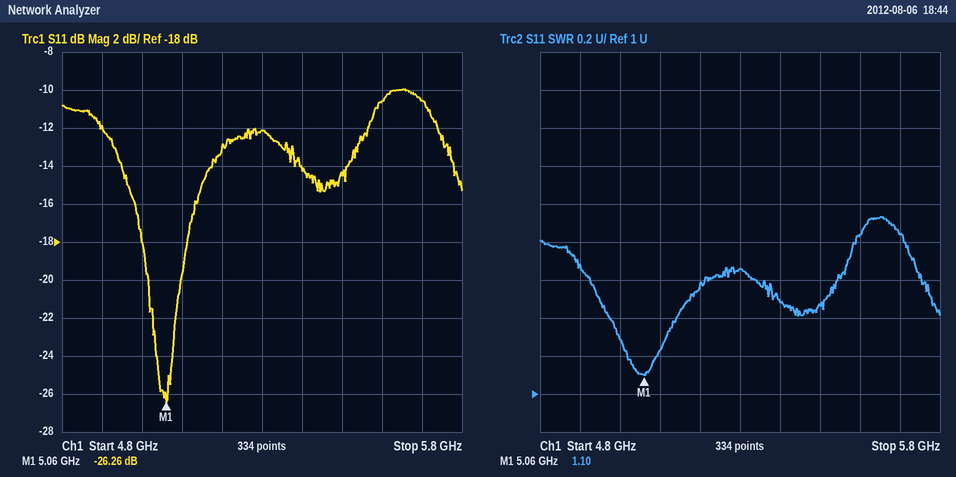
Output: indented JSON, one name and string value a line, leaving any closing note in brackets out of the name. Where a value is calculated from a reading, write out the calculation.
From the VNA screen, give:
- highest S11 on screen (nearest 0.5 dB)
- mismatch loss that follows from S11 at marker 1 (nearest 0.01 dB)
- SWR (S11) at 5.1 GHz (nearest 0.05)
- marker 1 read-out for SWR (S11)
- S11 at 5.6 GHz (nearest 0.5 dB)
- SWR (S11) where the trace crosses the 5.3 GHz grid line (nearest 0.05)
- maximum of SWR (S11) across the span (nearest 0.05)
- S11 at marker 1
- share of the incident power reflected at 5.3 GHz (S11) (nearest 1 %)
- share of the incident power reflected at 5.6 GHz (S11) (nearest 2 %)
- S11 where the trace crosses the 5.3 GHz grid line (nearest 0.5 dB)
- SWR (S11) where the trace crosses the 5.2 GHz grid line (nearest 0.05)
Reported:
{
  "highest S11 on screen": "-10.0 dB",
  "mismatch loss that follows from S11 at marker 1": "−10 log10(1 − 10^(-26.26/10)) ≈ 0.01 dB",
  "SWR (S11) at 5.1 GHz": "1.25",
  "marker 1 read-out for SWR": "1.10",
  "S11 at 5.6 GHz": "-10.5 dB",
  "SWR (S11) where the trace crosses the 5.3 GHz grid line": "1.65",
  "maximum of SWR (S11) across the span": "1.95",
  "S11 at marker 1": "-26.26 dB",
  "share of the incident power reflected at 5.3 GHz (S11)": "10^(-12/10) ≈ 6 %",
  "share of the incident power reflected at 5.6 GHz (S11)": "10^(-10.5/10) ≈ 8.91 %, so 8 % to the nearest 2 %",
  "S11 where the trace crosses the 5.3 GHz grid line": "-12.0 dB",
  "SWR (S11) where the trace crosses the 5.2 GHz grid line": "1.55"
}
